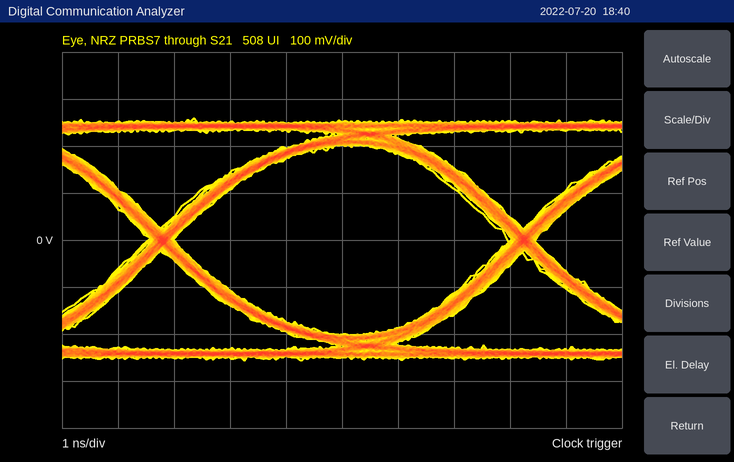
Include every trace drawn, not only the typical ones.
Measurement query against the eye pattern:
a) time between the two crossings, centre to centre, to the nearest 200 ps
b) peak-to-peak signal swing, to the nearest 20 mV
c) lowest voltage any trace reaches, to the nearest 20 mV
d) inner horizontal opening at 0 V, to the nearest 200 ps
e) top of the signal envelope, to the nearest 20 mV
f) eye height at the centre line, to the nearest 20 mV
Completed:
6.4 ns
520 mV
-260 mV
6.0 ns
260 mV
400 mV
